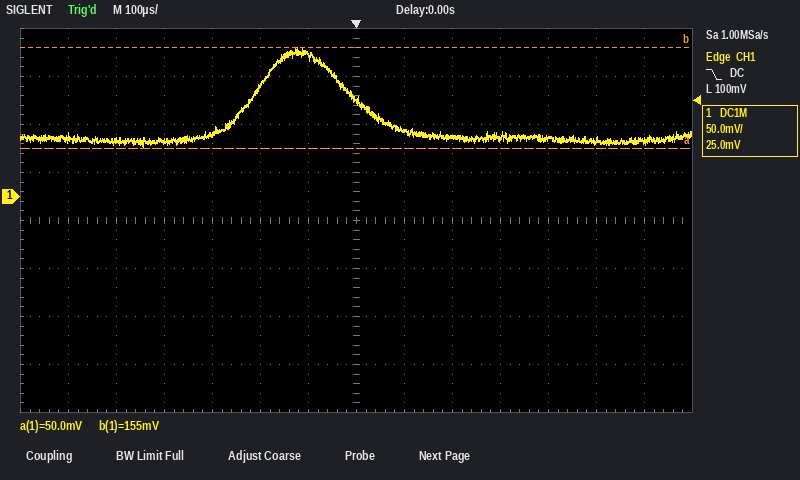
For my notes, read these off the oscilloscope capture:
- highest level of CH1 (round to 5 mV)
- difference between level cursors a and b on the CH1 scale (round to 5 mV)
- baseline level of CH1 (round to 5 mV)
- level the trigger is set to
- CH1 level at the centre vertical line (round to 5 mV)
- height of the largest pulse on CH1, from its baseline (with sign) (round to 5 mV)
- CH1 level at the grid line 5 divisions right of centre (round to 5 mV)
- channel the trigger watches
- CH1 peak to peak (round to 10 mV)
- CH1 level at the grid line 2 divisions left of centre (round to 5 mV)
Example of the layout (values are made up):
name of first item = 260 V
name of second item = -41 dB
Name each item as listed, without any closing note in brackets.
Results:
highest level of CH1 = 155 mV
difference between level cursors a and b on the CH1 scale = 105 mV
baseline level of CH1 = 60 mV
level the trigger is set to = 100 mV
CH1 level at the centre vertical line = 100 mV
height of the largest pulse on CH1, from its baseline (with sign) = +95 mV
CH1 level at the grid line 5 divisions right of centre = 60 mV
channel the trigger watches = CH1
CH1 peak to peak = 100 mV
CH1 level at the grid line 2 divisions left of centre = 115 mV
